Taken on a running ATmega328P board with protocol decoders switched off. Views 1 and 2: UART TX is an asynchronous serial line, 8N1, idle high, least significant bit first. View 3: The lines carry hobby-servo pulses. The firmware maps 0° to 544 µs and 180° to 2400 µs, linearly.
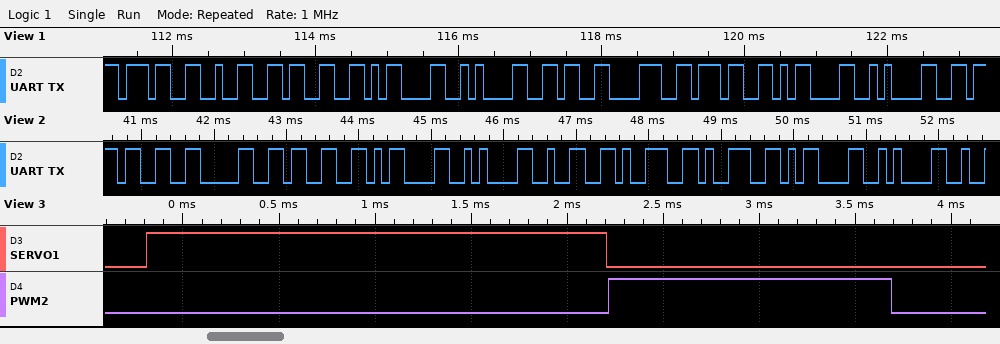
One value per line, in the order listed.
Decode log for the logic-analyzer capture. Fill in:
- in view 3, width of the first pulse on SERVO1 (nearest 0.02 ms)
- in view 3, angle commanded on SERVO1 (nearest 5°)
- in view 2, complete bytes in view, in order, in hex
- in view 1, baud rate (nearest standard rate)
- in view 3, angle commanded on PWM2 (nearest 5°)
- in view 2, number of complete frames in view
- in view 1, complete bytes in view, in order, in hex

2.40 ms
180°
0x33 0x30 0x33 0x0D 0x0A 0x32 0x39 0x39 0x0D 0x0A
9600 baud
90°
10
37 32 33 0D 0A 36 38 37 0D 0A
